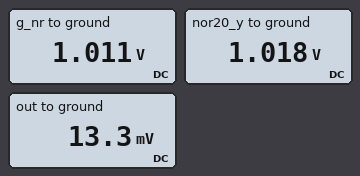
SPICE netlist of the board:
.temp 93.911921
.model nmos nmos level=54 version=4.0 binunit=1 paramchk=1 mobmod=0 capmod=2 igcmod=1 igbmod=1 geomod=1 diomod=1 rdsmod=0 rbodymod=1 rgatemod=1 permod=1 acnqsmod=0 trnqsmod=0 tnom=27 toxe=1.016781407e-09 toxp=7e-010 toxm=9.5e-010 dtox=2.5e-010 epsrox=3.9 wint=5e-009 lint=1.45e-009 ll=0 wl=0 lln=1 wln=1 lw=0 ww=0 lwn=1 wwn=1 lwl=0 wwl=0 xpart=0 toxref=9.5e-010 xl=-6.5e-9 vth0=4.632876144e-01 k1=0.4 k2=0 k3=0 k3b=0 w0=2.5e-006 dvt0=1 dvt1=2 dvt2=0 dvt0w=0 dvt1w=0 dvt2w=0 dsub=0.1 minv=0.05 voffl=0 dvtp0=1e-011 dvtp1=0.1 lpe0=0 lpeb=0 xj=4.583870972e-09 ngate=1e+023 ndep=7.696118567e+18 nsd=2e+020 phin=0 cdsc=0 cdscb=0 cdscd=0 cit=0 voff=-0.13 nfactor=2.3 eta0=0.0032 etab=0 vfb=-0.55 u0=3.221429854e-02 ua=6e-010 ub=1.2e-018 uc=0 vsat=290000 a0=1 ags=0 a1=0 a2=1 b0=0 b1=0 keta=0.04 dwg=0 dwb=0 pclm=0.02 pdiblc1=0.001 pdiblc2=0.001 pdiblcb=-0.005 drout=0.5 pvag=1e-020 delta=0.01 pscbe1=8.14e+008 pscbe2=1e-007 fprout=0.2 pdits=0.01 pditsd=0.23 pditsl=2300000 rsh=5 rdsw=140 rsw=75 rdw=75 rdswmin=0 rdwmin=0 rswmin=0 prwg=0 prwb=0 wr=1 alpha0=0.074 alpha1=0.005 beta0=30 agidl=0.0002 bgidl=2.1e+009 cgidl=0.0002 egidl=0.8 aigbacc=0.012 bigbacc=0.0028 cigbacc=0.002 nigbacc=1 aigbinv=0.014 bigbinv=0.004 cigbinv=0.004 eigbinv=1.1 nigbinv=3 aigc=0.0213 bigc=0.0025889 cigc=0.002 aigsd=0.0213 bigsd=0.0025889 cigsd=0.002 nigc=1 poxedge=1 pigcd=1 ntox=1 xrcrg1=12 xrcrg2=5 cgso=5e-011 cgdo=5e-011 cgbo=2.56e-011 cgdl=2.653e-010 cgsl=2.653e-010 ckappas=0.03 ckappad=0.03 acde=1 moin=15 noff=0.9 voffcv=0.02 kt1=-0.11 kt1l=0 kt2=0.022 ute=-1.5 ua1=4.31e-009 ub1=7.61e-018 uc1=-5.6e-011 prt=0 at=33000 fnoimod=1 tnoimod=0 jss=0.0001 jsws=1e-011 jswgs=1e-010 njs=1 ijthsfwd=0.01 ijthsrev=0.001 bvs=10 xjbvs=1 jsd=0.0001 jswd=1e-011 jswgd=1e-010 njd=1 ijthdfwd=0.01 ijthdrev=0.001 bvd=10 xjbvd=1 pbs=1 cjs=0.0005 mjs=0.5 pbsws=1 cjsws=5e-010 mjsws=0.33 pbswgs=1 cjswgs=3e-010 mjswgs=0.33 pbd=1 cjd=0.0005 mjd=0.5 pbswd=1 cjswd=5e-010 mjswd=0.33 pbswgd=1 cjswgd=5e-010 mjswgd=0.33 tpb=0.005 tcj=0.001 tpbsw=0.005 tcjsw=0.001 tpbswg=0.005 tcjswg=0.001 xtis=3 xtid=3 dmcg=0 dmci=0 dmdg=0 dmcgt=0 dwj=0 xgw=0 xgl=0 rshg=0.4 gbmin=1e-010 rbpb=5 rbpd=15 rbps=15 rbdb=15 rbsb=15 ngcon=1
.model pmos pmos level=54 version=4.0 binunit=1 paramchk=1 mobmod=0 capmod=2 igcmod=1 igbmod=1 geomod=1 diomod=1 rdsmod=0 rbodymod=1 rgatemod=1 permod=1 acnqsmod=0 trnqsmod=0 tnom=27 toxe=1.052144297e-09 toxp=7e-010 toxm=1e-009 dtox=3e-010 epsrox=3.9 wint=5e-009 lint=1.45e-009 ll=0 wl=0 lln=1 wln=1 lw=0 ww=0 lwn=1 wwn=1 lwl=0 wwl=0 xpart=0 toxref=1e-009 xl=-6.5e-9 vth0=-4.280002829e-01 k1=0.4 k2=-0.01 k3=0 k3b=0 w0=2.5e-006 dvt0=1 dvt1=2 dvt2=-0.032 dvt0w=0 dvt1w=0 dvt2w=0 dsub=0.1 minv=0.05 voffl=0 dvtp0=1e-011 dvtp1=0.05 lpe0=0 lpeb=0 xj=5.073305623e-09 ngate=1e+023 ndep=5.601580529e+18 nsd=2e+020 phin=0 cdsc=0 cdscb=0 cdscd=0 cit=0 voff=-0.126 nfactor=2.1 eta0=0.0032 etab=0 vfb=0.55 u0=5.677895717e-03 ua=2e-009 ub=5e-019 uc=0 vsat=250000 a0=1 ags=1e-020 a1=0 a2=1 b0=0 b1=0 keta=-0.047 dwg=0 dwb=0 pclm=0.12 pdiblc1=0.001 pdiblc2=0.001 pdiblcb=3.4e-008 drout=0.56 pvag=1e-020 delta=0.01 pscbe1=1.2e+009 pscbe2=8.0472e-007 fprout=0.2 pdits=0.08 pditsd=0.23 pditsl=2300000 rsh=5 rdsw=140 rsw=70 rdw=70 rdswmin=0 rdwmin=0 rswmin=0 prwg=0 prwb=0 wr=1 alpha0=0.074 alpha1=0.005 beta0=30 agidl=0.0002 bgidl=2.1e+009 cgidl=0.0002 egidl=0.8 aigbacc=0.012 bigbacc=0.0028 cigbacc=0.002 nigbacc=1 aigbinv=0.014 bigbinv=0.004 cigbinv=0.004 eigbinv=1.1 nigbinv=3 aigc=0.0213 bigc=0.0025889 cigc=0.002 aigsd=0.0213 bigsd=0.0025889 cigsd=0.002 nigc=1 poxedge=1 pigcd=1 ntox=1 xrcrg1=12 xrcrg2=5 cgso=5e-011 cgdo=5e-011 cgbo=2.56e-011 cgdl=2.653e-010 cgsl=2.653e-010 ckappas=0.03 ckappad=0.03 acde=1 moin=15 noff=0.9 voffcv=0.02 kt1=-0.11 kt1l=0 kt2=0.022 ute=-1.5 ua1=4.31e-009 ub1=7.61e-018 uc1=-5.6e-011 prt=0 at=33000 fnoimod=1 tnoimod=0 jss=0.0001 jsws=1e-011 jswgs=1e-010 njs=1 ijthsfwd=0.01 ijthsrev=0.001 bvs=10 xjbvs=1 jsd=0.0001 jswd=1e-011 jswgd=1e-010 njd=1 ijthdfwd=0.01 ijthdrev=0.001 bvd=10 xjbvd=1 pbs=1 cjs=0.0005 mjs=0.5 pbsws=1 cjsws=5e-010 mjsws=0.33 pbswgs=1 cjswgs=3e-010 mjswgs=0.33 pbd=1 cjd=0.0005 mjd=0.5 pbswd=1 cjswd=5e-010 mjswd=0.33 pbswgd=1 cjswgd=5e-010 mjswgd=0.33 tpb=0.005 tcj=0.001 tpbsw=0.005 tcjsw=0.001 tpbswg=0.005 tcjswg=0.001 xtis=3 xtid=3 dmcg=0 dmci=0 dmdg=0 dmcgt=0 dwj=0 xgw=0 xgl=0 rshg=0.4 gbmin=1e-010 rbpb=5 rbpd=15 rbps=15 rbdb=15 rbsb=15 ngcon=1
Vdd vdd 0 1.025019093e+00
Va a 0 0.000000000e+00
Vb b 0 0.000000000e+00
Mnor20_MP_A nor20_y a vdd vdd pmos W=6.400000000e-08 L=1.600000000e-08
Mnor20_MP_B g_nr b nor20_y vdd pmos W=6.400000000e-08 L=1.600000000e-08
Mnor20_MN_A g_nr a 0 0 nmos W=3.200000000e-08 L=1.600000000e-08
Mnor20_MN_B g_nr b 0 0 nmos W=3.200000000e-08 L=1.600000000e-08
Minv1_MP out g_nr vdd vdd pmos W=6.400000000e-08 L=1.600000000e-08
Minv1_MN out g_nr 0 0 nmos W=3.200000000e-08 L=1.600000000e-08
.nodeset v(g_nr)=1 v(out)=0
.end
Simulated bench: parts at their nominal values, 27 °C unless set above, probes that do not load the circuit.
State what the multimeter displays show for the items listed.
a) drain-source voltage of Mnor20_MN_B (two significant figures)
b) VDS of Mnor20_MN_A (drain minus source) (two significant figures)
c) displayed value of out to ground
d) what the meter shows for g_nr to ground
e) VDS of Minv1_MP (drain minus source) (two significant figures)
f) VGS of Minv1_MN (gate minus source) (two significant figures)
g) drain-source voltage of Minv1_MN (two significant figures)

1.0 V
1.0 V
13.3 mV
1.011 V
-1.0 V
1.0 V
13 mV
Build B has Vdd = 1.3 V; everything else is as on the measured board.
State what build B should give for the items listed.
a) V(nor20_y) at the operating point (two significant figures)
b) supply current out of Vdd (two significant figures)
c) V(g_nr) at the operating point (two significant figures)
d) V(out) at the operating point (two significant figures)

1.3 V
16 µA
1.2 V
120 mV
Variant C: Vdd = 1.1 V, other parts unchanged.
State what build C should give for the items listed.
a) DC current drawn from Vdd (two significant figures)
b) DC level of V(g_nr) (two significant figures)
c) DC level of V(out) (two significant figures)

3.9 µA
1.1 V
27 mV
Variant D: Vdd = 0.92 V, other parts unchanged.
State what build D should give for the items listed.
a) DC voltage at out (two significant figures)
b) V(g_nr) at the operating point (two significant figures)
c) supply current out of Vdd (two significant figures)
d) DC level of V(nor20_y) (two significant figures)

4.8 mV
910 mV
760 nA
920 mV
